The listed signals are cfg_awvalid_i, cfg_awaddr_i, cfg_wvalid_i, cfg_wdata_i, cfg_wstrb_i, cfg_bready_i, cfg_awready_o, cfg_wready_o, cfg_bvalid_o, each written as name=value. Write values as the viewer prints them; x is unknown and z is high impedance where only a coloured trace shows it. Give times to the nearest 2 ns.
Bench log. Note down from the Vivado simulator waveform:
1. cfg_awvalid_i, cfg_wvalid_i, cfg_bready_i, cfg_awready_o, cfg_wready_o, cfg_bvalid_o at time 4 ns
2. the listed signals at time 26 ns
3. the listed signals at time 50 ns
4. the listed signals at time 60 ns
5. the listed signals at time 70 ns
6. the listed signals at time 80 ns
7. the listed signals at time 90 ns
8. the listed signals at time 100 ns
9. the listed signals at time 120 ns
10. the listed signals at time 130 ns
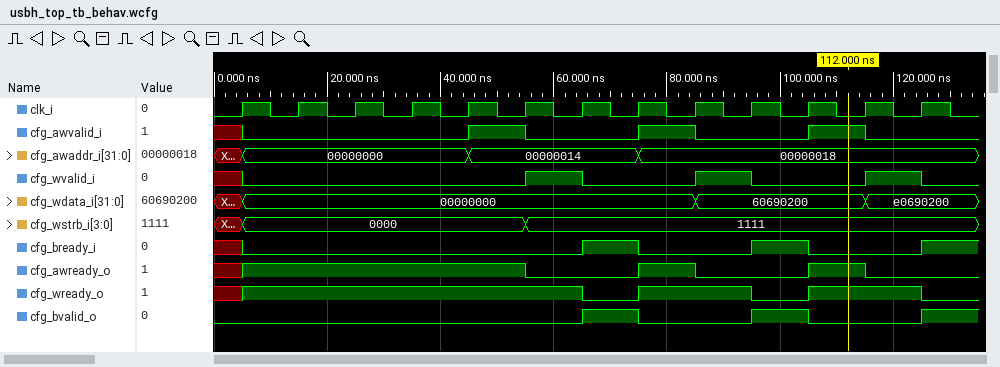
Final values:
cfg_awvalid_i=x, cfg_wvalid_i=x, cfg_bready_i=x, cfg_awready_o=x, cfg_wready_o=x, cfg_bvalid_o=0
cfg_awvalid_i=0, cfg_awaddr_i=00000000, cfg_wvalid_i=0, cfg_wdata_i=00000000, cfg_wstrb_i=0000, cfg_bready_i=0, cfg_awready_o=1, cfg_wready_o=1, cfg_bvalid_o=0
cfg_awvalid_i=1, cfg_awaddr_i=00000014, cfg_wvalid_i=0, cfg_wdata_i=00000000, cfg_wstrb_i=0000, cfg_bready_i=0, cfg_awready_o=1, cfg_wready_o=1, cfg_bvalid_o=0
cfg_awvalid_i=0, cfg_awaddr_i=00000014, cfg_wvalid_i=1, cfg_wdata_i=00000000, cfg_wstrb_i=1111, cfg_bready_i=0, cfg_awready_o=0, cfg_wready_o=1, cfg_bvalid_o=0
cfg_awvalid_i=0, cfg_awaddr_i=00000014, cfg_wvalid_i=0, cfg_wdata_i=00000000, cfg_wstrb_i=1111, cfg_bready_i=1, cfg_awready_o=0, cfg_wready_o=0, cfg_bvalid_o=1
cfg_awvalid_i=1, cfg_awaddr_i=00000018, cfg_wvalid_i=0, cfg_wdata_i=00000000, cfg_wstrb_i=1111, cfg_bready_i=0, cfg_awready_o=1, cfg_wready_o=1, cfg_bvalid_o=0
cfg_awvalid_i=0, cfg_awaddr_i=00000018, cfg_wvalid_i=1, cfg_wdata_i=60690200, cfg_wstrb_i=1111, cfg_bready_i=0, cfg_awready_o=0, cfg_wready_o=1, cfg_bvalid_o=0
cfg_awvalid_i=0, cfg_awaddr_i=00000018, cfg_wvalid_i=0, cfg_wdata_i=60690200, cfg_wstrb_i=1111, cfg_bready_i=1, cfg_awready_o=0, cfg_wready_o=0, cfg_bvalid_o=1
cfg_awvalid_i=0, cfg_awaddr_i=00000018, cfg_wvalid_i=1, cfg_wdata_i=e0690200, cfg_wstrb_i=1111, cfg_bready_i=0, cfg_awready_o=0, cfg_wready_o=1, cfg_bvalid_o=0
cfg_awvalid_i=0, cfg_awaddr_i=00000018, cfg_wvalid_i=0, cfg_wdata_i=e0690200, cfg_wstrb_i=1111, cfg_bready_i=1, cfg_awready_o=0, cfg_wready_o=0, cfg_bvalid_o=1
